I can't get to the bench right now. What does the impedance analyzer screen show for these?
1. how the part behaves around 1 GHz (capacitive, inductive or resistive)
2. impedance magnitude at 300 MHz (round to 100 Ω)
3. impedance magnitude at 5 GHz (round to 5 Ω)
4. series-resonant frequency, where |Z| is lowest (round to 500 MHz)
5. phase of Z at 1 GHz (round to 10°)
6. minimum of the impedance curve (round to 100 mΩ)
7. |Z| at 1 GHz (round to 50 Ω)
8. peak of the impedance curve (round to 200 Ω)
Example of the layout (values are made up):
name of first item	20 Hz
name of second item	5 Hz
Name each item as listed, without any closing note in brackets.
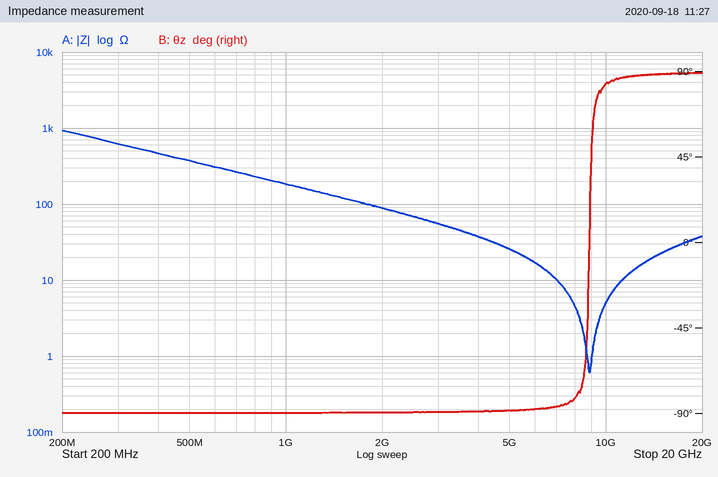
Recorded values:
how the part behaves around 1 GHz	capacitive
impedance magnitude at 300 MHz	600 Ω
impedance magnitude at 5 GHz	25 Ω
series-resonant frequency, where |Z| is lowest	9.0 GHz
phase of Z at 1 GHz	-90°
minimum of the impedance curve	600 mΩ
|Z| at 1 GHz	200 Ω
peak of the impedance curve	1.0 kΩ
